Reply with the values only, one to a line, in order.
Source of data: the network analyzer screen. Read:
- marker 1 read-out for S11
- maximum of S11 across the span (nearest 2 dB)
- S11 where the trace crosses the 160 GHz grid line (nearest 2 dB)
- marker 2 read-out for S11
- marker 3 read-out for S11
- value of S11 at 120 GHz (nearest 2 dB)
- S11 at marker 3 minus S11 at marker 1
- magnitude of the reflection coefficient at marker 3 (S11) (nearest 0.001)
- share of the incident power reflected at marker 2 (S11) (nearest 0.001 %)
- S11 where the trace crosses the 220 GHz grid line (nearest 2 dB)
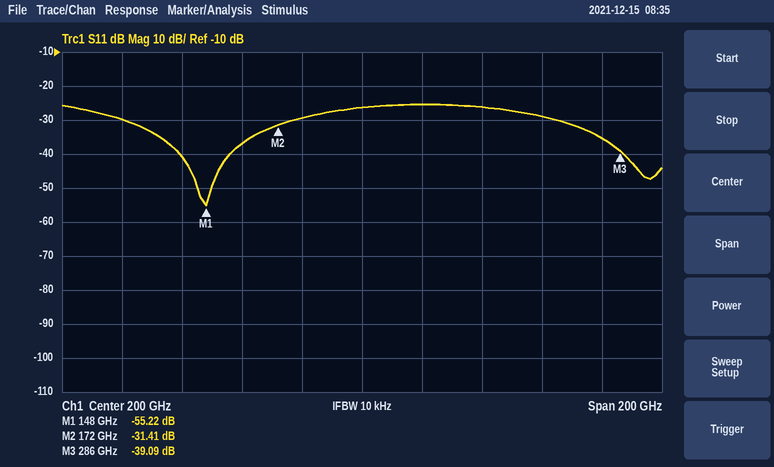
-55.22 dB
-26 dB
-36 dB
-31.41 dB
-39.09 dB
-30 dB
16.13 dB
0.011
0.072 %
-26 dB
